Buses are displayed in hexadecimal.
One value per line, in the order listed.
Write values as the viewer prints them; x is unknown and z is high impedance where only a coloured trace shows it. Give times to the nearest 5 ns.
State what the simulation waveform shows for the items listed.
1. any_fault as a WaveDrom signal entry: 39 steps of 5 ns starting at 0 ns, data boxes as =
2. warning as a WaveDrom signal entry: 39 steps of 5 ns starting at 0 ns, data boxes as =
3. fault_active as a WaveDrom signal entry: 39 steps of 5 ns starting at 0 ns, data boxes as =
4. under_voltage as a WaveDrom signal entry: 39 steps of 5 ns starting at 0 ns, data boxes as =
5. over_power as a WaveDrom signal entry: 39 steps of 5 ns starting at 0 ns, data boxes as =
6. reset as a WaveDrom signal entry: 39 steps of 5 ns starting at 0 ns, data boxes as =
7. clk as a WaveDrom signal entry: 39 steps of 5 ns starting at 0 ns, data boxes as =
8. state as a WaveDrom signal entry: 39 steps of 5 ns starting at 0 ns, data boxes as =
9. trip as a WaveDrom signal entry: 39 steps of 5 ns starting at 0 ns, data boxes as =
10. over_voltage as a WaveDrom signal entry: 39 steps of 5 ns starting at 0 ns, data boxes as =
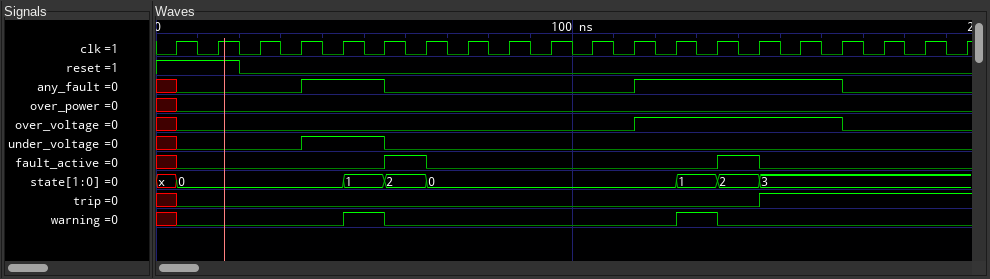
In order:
{name: 'any_fault', wave: 'x0.....1...0...........1.........0.....'}
{name: 'warning', wave: 'x0.......1.0.............1.0...........'}
{name: 'fault_active', wave: 'x0.........1.0.............1.0.........'}
{name: 'under_voltage', wave: 'x0.....1...0...........................'}
{name: 'over_power', wave: 'x0.....................................'}
{name: 'reset', wave: '1...0..................................'}
{name: 'clk', wave: '010101010101010101010101010101010101010'}
{name: 'state', wave: 'x=.......=.=.=...........=.=.=.........', data: '0 1 2 0 1 2 3'}
{name: 'trip', wave: 'x0...........................1.........'}
{name: 'over_voltage', wave: 'x0.....................1.........0.....'}
